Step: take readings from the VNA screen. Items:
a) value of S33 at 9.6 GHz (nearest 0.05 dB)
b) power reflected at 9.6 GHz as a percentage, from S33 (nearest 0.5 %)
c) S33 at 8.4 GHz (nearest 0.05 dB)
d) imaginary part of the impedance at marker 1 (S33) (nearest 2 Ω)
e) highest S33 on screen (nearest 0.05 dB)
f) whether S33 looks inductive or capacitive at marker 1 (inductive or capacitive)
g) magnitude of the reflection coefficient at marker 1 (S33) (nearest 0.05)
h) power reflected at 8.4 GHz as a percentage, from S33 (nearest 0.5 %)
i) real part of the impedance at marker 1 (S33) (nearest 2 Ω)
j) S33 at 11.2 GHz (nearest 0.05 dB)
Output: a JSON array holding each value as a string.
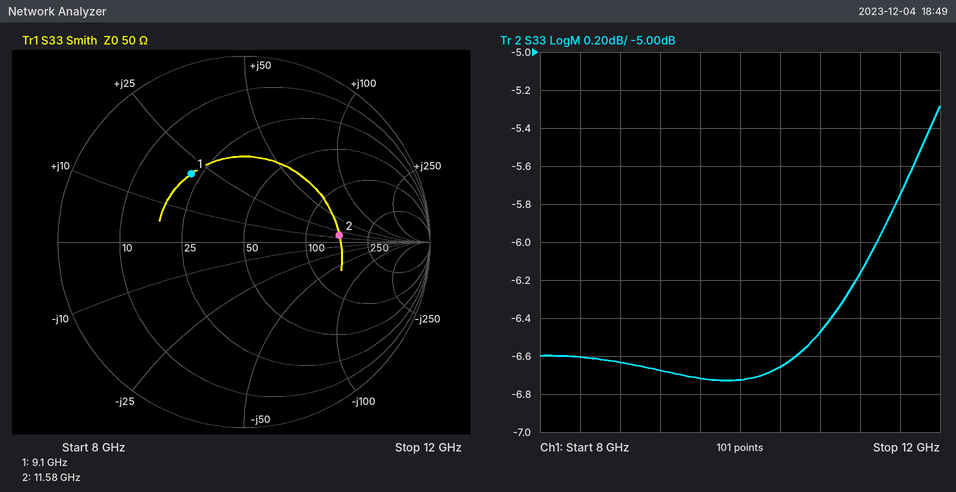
["-6.70 dB", "21.5 %", "-6.60 dB", "+20 Ω", "-5.30 dB", "inductive", "0.45", "22.0 %", "22 Ω", "-6.15 dB"]
